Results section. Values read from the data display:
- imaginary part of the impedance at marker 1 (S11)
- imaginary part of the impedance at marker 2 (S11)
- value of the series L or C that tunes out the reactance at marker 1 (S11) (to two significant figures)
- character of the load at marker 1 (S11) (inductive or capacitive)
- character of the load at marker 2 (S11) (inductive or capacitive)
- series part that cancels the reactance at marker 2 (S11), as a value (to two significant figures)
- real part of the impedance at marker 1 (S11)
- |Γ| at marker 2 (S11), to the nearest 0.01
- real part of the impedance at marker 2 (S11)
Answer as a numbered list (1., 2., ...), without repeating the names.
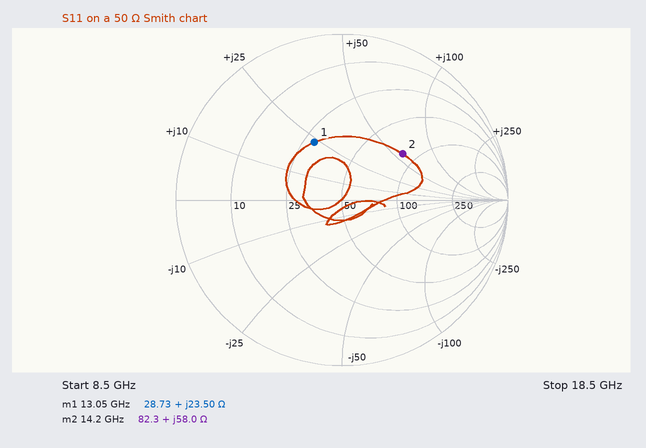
1. +23.50 Ω
2. +58.0 Ω
3. 520 fF
4. inductive
5. inductive
6. 190 fF
7. 28.73 Ω
8. 0.46
9. 82.3 Ω
